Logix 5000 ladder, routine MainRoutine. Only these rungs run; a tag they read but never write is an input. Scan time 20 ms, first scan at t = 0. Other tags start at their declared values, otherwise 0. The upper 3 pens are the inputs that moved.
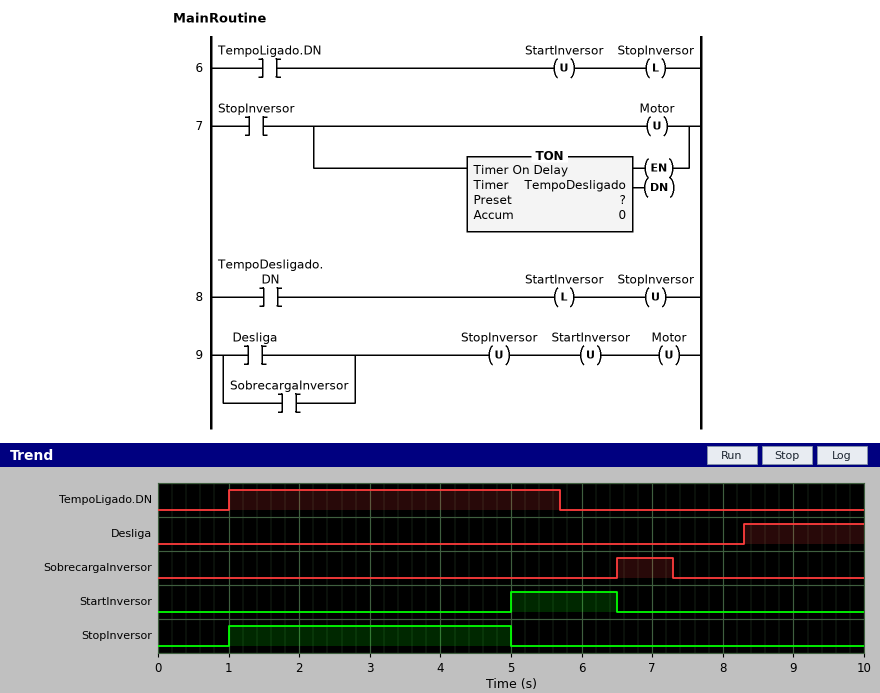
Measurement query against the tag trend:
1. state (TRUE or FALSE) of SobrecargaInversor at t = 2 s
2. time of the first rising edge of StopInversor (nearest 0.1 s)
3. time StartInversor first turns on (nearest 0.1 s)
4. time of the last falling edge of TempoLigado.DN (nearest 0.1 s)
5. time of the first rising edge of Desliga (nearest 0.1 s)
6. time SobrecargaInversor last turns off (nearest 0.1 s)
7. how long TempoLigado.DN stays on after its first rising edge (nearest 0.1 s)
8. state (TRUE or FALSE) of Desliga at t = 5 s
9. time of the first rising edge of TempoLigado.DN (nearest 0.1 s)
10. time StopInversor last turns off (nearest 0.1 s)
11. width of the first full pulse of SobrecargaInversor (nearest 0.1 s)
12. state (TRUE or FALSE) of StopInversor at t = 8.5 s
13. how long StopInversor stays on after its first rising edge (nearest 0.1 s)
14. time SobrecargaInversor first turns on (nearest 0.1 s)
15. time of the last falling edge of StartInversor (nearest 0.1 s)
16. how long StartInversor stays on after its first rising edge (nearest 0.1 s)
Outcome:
FALSE
1.0 s
5.0 s
5.7 s
8.3 s
7.3 s
4.7 s
FALSE
1.0 s
5.0 s
0.8 s
FALSE
4.0 s
6.5 s
6.5 s
1.5 s
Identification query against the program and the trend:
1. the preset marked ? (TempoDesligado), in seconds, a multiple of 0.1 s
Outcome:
4.0 s
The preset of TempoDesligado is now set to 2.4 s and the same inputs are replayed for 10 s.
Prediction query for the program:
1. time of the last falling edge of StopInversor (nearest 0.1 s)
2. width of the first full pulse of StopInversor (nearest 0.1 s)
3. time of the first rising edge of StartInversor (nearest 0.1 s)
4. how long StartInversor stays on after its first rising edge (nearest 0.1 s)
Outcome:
3.4 s
2.4 s
3.4 s
3.1 s
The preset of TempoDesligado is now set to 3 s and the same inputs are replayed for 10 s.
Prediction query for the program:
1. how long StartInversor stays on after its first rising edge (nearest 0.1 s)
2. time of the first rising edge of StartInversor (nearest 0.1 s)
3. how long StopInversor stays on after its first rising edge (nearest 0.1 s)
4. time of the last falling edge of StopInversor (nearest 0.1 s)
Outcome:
2.5 s
4.0 s
3.0 s
4.0 s
